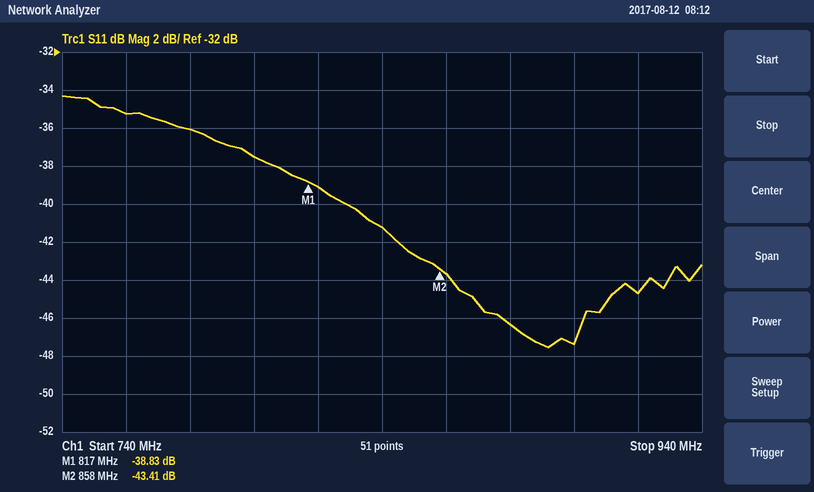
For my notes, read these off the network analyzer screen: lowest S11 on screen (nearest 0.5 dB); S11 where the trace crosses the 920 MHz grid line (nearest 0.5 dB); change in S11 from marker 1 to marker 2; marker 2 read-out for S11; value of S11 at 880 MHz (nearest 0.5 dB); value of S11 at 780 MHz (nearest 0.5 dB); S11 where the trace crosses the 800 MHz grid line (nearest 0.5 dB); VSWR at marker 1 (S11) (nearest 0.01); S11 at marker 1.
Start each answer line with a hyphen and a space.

- -47.5 dB
- -44.5 dB
- -4.58 dB
- -43.41 dB
- -46.5 dB
- -36.0 dB
- -37.5 dB
- 1.02
- -38.83 dB
